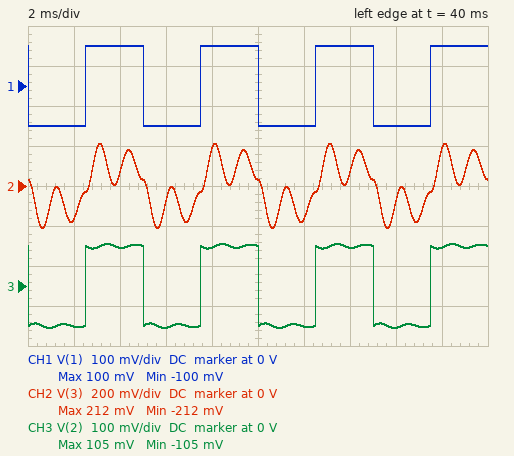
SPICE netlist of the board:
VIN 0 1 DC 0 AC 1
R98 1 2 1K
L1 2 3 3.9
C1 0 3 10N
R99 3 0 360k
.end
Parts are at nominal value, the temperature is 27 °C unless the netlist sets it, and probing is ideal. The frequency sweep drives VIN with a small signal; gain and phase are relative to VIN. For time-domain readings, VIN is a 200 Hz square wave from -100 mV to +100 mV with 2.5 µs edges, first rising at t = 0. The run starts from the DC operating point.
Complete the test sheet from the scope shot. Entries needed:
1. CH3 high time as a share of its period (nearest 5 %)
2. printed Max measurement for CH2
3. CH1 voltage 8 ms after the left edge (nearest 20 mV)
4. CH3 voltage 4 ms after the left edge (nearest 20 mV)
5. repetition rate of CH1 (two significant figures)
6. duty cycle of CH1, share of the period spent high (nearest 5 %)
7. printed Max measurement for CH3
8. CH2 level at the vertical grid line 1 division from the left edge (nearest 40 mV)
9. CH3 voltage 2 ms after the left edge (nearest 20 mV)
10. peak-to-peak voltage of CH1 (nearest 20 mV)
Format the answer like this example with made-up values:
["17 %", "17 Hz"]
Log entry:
["50 %", "212 mV", "100 mV", "100 mV", "200 Hz", "50 %", "105 mV", "-160 mV", "-100 mV", "200 mV"]
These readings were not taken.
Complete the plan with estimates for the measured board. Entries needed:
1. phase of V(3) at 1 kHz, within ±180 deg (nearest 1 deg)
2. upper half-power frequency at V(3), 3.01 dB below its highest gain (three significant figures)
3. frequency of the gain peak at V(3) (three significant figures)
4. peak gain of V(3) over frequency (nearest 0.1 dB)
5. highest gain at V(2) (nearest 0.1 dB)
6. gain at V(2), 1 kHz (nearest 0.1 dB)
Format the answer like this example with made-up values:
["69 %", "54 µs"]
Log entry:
["14 deg", "846 Hz", "805 Hz", "19.5 dB", "0 dB", "-0.1 dB"]
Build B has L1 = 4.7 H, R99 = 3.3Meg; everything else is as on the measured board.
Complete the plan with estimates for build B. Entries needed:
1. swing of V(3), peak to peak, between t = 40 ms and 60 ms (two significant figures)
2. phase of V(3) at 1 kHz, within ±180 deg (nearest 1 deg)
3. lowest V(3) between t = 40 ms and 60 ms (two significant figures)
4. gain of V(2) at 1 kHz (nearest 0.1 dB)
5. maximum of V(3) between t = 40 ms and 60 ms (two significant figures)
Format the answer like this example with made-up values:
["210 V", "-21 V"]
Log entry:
["450 mV", "5 deg", "-220 mV", "0 dB", "220 mV"]
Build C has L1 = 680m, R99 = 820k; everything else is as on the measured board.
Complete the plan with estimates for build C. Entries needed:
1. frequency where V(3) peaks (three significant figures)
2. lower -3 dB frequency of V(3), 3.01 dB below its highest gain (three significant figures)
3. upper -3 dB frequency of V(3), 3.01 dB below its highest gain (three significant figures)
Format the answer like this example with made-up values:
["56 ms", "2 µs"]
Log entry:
["1.92 kHz", "1.79 kHz", "2.05 kHz"]
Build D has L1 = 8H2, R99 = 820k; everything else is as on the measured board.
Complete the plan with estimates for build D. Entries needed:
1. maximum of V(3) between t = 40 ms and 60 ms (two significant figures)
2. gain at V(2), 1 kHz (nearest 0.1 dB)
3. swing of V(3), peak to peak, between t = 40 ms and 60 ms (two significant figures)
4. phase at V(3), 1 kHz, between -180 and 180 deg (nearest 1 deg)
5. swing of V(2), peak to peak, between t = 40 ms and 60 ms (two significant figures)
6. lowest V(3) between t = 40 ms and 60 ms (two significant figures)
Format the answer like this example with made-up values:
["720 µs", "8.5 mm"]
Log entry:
["370 mV", "0 dB", "740 mV", "3 deg", "220 mV", "-370 mV"]
